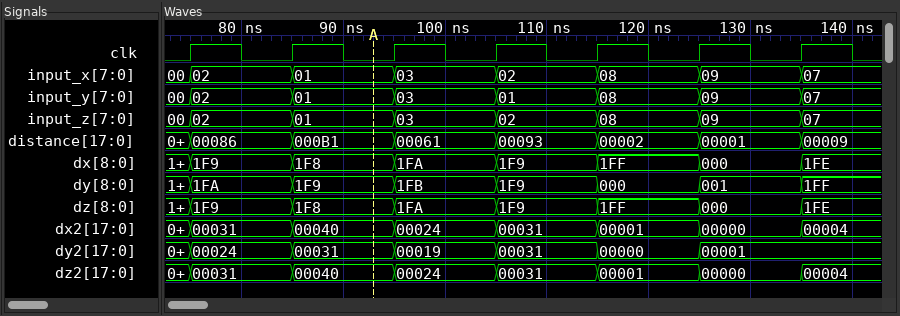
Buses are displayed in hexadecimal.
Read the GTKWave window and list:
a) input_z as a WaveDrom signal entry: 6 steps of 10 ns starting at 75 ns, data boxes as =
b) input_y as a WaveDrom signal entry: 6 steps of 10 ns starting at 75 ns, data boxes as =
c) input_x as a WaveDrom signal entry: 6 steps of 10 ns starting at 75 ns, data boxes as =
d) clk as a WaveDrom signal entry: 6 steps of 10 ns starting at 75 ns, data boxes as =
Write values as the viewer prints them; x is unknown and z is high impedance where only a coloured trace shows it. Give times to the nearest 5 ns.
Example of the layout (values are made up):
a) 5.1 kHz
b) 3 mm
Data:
a) {name: 'input_z', wave: '======', data: '02 01 03 02 08 09'}
b) {name: 'input_y', wave: '======', data: '02 01 03 01 08 09'}
c) {name: 'input_x', wave: '======', data: '02 01 03 02 08 09'}
d) {name: 'clk', wave: 'p.....'}
